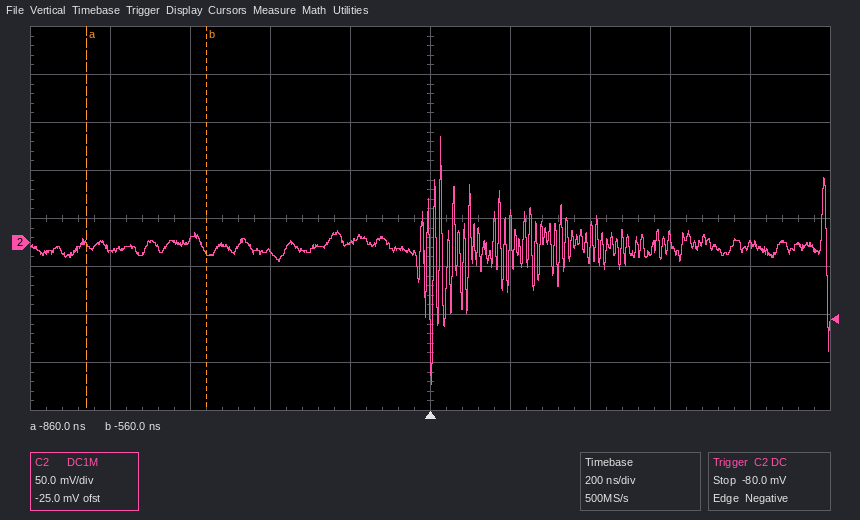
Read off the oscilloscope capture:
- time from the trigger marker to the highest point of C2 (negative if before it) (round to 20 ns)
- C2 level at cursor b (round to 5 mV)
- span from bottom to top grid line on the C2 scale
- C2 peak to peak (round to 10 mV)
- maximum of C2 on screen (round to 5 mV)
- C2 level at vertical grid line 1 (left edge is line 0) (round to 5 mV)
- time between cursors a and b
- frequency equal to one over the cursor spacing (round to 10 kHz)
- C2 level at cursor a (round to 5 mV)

+20 ns
-10 mV
400 mV
260 mV
110 mV
-5 mV
300 ns
3.33 MHz
0 mV
